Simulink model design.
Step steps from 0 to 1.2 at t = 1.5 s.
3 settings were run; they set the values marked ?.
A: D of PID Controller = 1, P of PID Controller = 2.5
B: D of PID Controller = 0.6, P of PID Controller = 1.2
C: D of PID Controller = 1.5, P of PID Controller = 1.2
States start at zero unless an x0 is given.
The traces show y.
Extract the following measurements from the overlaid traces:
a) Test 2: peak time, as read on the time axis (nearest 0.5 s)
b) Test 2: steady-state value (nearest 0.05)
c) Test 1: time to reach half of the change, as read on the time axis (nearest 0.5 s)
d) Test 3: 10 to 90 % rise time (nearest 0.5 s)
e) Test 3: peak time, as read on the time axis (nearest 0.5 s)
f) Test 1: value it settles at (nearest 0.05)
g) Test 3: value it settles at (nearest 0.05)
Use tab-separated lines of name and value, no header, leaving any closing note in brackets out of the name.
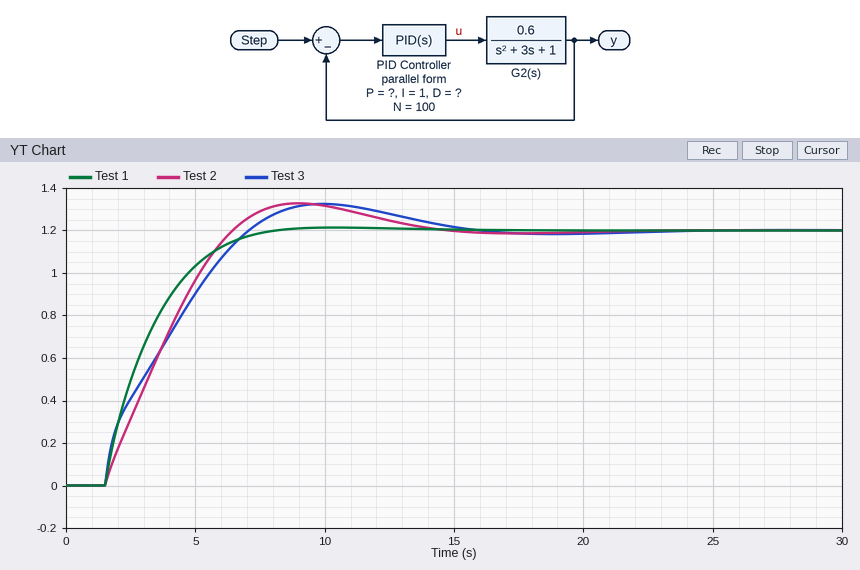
Test 2: peak time, as read on the time axis	9.0 s
Test 2: steady-state value	1.20
Test 1: time to reach half of the change, as read on the time axis	3.0 s
Test 3: 10 to 90 % rise time	4.5 s
Test 3: peak time, as read on the time axis	10.0 s
Test 1: value it settles at	1.20
Test 3: value it settles at	1.20
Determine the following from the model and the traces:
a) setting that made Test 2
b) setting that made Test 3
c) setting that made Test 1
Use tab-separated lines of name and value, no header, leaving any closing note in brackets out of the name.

setting that made Test 2	B
setting that made Test 3	C
setting that made Test 1	A
